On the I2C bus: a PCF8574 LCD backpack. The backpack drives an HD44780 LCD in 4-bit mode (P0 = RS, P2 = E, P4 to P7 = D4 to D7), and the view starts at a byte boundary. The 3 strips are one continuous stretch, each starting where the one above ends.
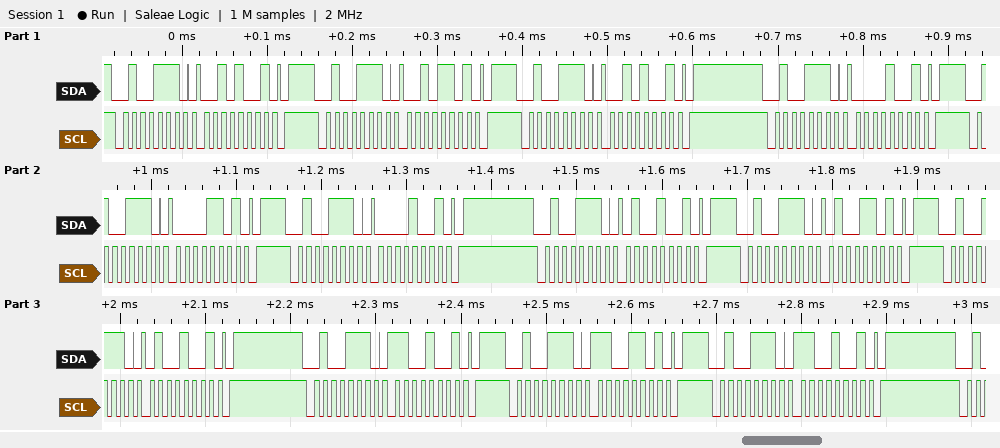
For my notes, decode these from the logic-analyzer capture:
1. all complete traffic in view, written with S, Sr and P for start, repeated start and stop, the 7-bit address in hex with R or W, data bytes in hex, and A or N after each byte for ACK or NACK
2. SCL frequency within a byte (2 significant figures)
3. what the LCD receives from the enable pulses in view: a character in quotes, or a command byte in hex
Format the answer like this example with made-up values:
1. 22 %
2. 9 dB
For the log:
1. S 27W A 29 A P S 27W A 2D A P S 27W A 29 A P S 27W A 09 A P S 27W A 0D A P S 27W A 09 A P S 27W A 49 A P S 27W A 4D A P S 27W A 49 A P S 27W A C9 A P S 27W A CD A P S 27W A C9 A P
2. 100 kHz
3. ' ' 'L'
